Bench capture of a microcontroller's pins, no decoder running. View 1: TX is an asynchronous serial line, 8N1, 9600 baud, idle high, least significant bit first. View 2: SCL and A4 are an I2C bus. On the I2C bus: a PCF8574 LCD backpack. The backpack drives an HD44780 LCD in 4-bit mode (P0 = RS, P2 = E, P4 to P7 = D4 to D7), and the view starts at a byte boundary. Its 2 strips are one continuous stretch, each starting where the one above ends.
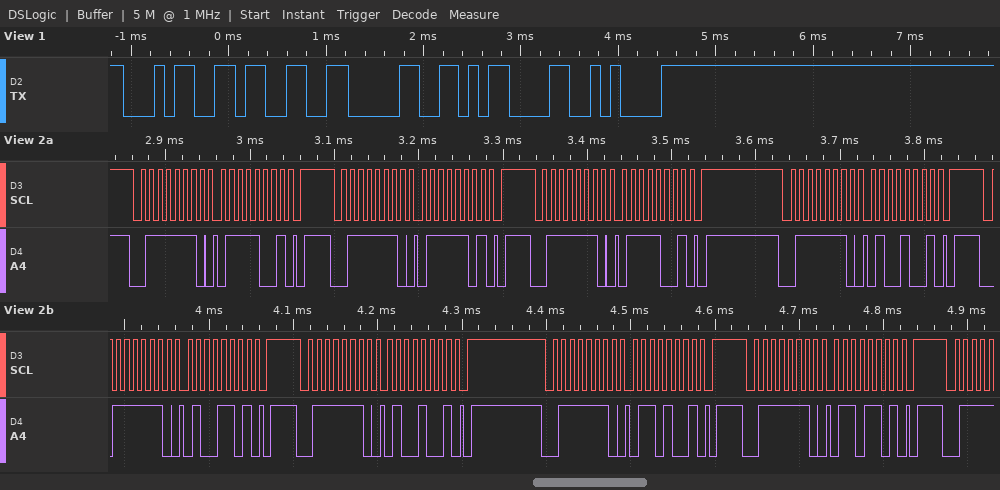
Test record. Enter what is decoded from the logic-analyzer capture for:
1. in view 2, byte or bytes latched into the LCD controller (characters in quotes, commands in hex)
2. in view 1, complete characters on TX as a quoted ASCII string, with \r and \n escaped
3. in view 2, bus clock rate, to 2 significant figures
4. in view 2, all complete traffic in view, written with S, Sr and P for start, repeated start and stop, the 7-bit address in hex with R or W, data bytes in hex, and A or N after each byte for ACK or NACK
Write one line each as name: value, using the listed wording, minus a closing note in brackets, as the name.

in view 2, byte or bytes latched into the LCD controller: 't'
in view 1, complete characters on TX as a quoted ASCII string, with \r and \n escaped: "430\r\n"
in view 2, bus clock rate, to 2 significant figures: 100 kHz
in view 2, all complete traffic in view, written with S, Sr and P for start, repeated start and stop, the 7-bit address in hex with R or W, data bytes in hex, and A or N after each byte for ACK or NACK: S 3FW A 79 A P S 3FW A 7D A P S 3FW A 79 A P S 3FW A 49 A P S 3FW A 4D A P S 3FW A 49 A P S 3FW A 69 A P S 3FW A 6D A P
